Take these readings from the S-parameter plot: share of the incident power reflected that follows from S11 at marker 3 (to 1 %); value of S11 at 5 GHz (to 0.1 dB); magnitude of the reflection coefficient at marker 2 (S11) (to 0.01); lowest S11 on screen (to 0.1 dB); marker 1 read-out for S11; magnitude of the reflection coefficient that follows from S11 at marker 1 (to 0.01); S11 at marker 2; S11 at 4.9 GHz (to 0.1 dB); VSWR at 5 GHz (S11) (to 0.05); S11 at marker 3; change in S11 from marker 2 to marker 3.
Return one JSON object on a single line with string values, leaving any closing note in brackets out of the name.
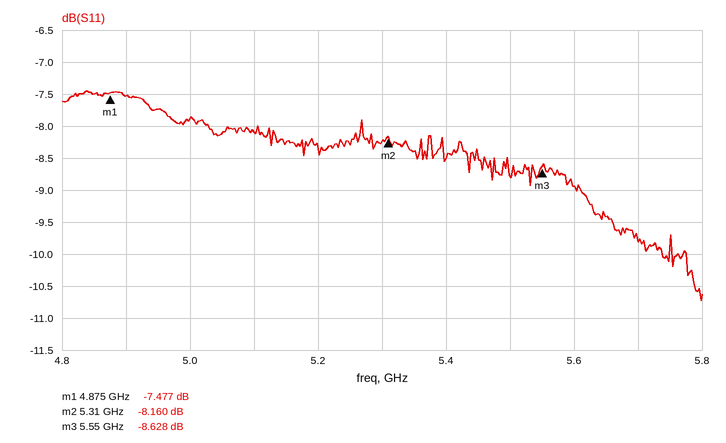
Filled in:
{"share of the incident power reflected that follows from S11 at marker 3": "14 %", "value of S11 at 5 GHz": "-7.9 dB", "magnitude of the reflection coefficient at marker 2 (S11)": "0.39", "lowest S11 on screen": "-10.7 dB", "marker 1 read-out for S11": "-7.477 dB", "magnitude of the reflection coefficient that follows from S11 at marker 1": "0.42", "S11 at marker 2": "-8.160 dB", "S11 at 4.9 GHz": "-7.5 dB", "VSWR at 5 GHz (S11)": "2.35", "S11 at marker 3": "-8.628 dB", "change in S11 from marker 2 to marker 3": "-0.468 dB"}
